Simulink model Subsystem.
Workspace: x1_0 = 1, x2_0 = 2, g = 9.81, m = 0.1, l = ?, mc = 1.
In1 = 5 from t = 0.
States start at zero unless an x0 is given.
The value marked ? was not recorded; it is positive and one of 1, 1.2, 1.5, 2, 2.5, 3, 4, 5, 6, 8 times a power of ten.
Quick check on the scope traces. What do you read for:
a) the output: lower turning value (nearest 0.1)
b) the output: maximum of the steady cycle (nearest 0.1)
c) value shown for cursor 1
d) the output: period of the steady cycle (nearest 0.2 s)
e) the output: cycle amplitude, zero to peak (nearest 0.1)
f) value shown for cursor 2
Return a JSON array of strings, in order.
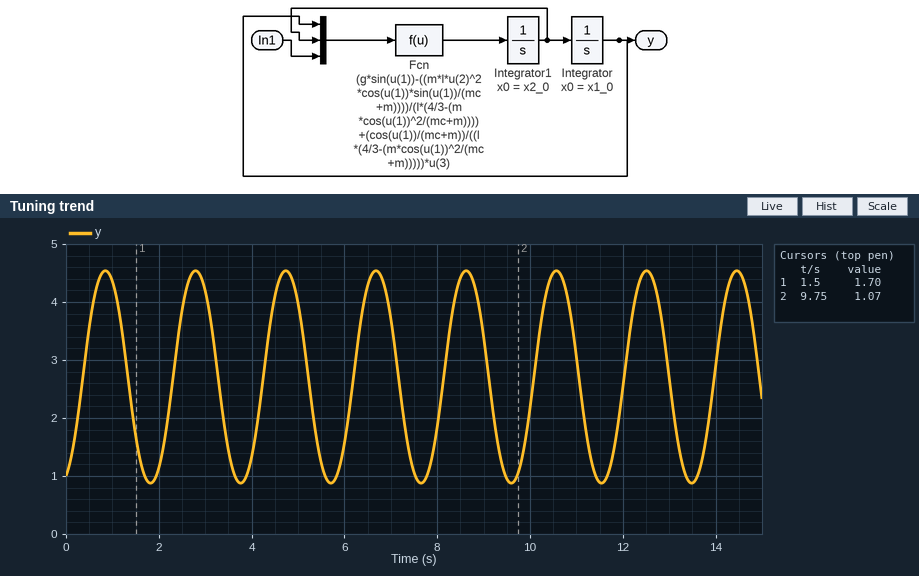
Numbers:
["0.9", "4.5", "1.70", "2.0 s", "1.8", "1.07"]
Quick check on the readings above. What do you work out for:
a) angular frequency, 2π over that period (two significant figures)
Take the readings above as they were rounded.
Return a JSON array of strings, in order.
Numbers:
["3.1 rad/s"]
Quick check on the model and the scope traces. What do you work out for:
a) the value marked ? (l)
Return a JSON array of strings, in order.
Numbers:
["0.5"]
